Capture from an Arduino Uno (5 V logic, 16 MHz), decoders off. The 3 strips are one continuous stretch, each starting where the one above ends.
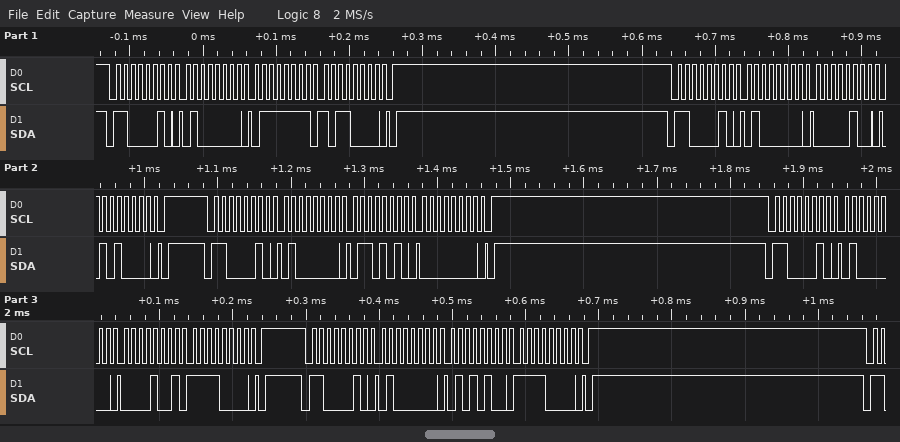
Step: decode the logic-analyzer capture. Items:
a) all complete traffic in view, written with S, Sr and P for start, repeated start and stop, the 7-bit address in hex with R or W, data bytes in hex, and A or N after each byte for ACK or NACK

S 61W A 40 A 7F A B0 A P S 61W A 40 A 04 A 50 A P S 61W A 40 A 6A A 00 A P S 61W A 40 A 09 A F0 A P S 61W A 40 A 54 A F0 A P
